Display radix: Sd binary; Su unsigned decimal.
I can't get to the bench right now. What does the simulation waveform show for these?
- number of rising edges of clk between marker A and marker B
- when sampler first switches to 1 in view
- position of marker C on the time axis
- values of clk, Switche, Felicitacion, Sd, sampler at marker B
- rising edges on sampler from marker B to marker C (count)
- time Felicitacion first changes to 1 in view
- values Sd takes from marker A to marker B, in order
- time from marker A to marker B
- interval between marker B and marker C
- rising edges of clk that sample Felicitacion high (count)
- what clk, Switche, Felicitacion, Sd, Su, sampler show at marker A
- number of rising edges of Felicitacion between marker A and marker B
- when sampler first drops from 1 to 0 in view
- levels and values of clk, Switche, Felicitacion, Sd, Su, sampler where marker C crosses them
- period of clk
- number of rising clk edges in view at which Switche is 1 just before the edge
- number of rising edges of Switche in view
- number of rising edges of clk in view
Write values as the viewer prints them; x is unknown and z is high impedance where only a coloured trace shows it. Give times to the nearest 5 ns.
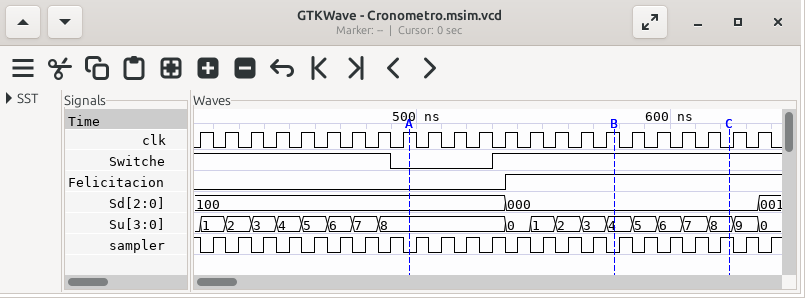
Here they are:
8
420 ns
625 ns
clk=1, Switche=1, Felicitacion=1, Sd=000, sampler=0
5
535 ns
100, 000
80 ns
45 ns
10
clk=1, Switche=0, Felicitacion=0, Sd=100, Su=8, sampler=0
1
415 ns
clk=0, Switche=1, Felicitacion=1, Sd=000, Su=8, sampler=1
10 ns
19
1
23
